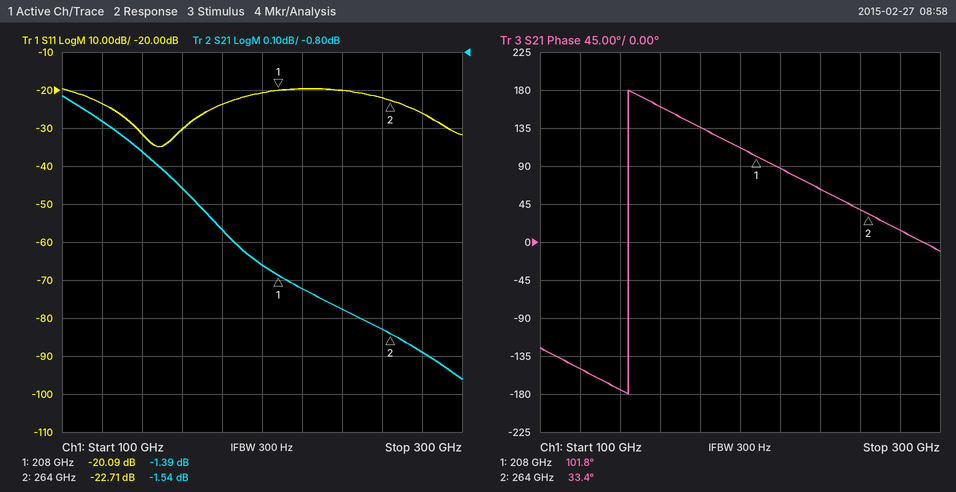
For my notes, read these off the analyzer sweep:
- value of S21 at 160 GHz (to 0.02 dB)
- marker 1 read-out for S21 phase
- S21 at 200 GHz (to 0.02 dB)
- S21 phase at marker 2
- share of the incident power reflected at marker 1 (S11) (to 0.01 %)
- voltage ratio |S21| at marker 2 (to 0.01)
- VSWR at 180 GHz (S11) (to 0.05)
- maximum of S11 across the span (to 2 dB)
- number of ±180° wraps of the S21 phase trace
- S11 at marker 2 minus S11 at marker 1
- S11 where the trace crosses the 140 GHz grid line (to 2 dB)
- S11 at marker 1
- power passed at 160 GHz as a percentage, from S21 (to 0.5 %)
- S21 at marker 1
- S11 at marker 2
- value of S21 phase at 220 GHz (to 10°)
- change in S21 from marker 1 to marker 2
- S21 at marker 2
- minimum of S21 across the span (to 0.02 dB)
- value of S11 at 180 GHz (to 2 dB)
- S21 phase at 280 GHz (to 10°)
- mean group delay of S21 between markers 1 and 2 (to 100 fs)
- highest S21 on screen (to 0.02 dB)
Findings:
-1.16 dB
101.8°
-1.36 dB
33.4°
0.98 %
0.84
1.15
-20 dB
1
-2.62 dB
-32 dB
-20.09 dB
76.5 %
-1.39 dB
-22.71 dB
90°
-0.15 dB
-1.54 dB
-1.66 dB
-24 dB
10°
3.4 ps
-0.92 dB
